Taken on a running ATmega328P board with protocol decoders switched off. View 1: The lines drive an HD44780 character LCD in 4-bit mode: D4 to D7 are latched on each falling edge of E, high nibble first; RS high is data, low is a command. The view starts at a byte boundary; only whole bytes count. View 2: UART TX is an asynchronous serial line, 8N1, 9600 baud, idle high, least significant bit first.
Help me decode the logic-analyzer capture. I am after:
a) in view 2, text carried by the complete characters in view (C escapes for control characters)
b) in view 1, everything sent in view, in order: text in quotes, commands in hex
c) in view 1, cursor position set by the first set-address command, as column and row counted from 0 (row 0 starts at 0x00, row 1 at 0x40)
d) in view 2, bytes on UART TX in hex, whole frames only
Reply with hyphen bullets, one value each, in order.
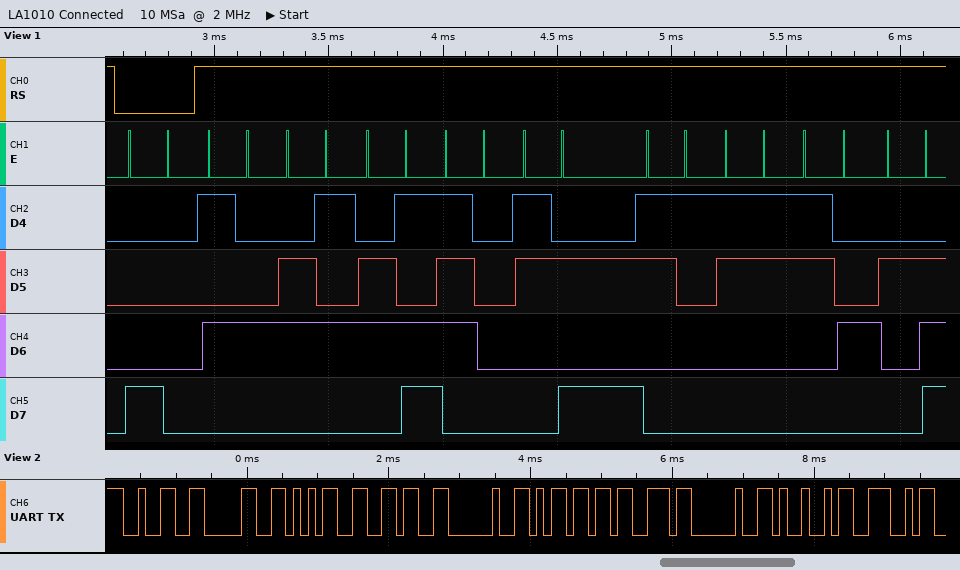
- "2056 ms IN"
- 0x80 "Temp:134."
- column 0, row 0
- 32 30 35 36 20 6D 73 20 49 4E
